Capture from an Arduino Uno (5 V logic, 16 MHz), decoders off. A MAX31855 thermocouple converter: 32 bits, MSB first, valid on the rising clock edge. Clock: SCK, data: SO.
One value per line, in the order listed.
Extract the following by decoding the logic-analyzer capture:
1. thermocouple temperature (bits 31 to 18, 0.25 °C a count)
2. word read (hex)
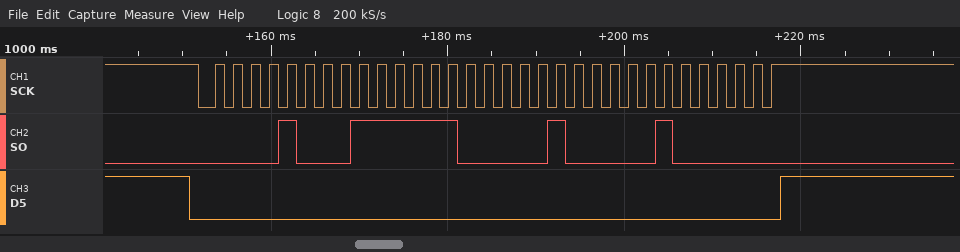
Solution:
143.75 °C
0x08FC1040
